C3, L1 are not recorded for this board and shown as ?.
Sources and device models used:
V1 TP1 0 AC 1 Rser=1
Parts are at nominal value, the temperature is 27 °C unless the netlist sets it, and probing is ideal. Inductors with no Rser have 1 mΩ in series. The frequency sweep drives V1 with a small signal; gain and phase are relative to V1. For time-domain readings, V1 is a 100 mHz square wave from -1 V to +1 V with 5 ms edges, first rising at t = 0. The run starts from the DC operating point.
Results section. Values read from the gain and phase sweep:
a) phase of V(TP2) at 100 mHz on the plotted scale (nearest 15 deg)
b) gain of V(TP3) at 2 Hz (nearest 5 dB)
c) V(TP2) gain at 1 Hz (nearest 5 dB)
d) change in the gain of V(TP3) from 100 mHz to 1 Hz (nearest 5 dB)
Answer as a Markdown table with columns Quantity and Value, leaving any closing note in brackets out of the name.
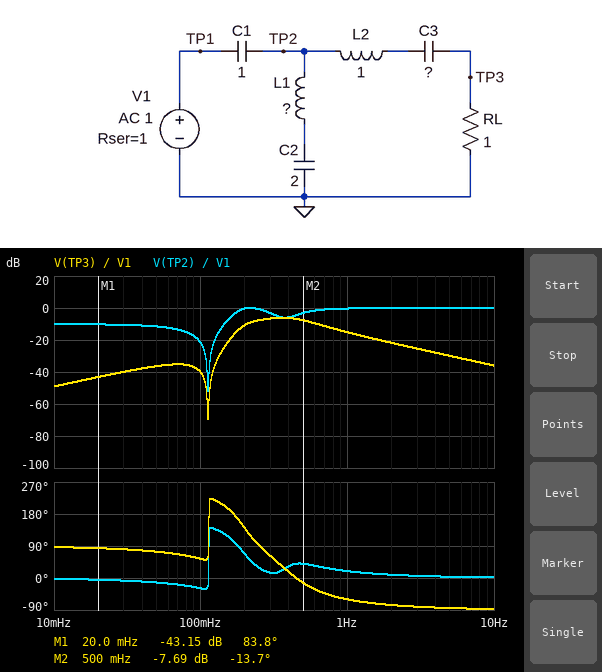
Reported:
| Quantity | Value |
|---|---|
| phase of V(TP2) at 100 mHz on the plotted scale | -30 deg |
| gain of V(TP3) at 2 Hz | -20 dB |
| V(TP2) gain at 1 Hz | 0 dB |
| change in the gain of V(TP3) from 100 mHz to 1 Hz | 25 dB |
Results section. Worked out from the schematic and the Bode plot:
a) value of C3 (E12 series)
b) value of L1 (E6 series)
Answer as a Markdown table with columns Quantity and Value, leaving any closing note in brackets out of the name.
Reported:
| Quantity | Value |
|---|---|
| value of C3 | 180 mF |
| value of L1 | 1 H |
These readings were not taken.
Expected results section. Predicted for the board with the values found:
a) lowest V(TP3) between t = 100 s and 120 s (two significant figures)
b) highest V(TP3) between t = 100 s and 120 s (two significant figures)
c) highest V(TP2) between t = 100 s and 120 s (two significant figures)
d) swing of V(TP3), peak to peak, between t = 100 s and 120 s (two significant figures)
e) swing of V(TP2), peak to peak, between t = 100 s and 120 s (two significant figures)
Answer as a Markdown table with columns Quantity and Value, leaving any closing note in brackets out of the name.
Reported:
| Quantity | Value |
|---|---|
| lowest V(TP3) between t = 100 s and 120 s | -390 mV |
| highest V(TP3) between t = 100 s and 120 s | 390 mV |
| highest V(TP2) between t = 100 s and 120 s | 1.8 V |
| swing of V(TP3), peak to peak, between t = 100 s and 120 s | 780 mV |
| swing of V(TP2), peak to peak, between t = 100 s and 120 s | 2.9 V |
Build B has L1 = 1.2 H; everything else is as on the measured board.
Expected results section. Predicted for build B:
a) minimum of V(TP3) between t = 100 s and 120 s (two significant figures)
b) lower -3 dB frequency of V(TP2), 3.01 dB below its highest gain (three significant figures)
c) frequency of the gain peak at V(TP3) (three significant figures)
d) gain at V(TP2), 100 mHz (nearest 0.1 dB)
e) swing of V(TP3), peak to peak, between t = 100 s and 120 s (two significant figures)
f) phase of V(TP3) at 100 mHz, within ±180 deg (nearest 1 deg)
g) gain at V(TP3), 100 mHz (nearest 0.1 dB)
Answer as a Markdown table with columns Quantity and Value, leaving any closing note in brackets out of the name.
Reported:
| Quantity | Value |
|---|---|
| minimum of V(TP3) between t = 100 s and 120 s | -380 mV |
| lower -3 dB frequency of V(TP2), 3.01 dB below its highest gain | 159 mHz |
| frequency of the gain peak at V(TP3) | 374 mHz |
| gain at V(TP2), 100 mHz | -33.3 dB |
| swing of V(TP3), peak to peak, between t = 100 s and 120 s | 760 mV |
| phase of V(TP3) at 100 mHz, within ±180 deg | 53 deg |
| gain at V(TP3), 100 mHz | -51.6 dB |
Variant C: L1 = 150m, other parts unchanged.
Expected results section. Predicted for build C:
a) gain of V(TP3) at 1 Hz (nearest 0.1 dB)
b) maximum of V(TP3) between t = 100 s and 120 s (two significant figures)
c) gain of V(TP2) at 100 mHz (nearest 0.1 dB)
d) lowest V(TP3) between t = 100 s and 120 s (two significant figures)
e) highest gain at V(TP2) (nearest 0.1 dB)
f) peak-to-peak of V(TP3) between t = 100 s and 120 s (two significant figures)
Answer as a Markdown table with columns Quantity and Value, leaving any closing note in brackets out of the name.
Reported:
| Quantity | Value |
|---|---|
| gain of V(TP3) at 1 Hz | -18.7 dB |
| maximum of V(TP3) between t = 100 s and 120 s | 150 mV |
| gain of V(TP2) at 100 mHz | -11.6 dB |
| lowest V(TP3) between t = 100 s and 120 s | -150 mV |
| highest gain at V(TP2) | 0 dB |
| peak-to-peak of V(TP3) between t = 100 s and 120 s | 310 mV |
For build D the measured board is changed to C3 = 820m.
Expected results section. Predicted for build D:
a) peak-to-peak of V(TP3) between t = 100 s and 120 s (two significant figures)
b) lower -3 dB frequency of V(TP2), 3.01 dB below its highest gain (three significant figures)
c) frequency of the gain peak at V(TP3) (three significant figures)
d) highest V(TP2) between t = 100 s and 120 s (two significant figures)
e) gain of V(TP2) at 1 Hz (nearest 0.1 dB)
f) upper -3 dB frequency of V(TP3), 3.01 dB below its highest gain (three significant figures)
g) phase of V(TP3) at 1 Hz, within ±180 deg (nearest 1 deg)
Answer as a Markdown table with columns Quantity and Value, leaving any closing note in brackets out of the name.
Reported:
| Quantity | Value |
|---|---|
| peak-to-peak of V(TP3) between t = 100 s and 120 s | 650 mV |
| lower -3 dB frequency of V(TP2), 3.01 dB below its highest gain | 333 mHz |
| frequency of the gain peak at V(TP3) | 233 mHz |
| highest V(TP2) between t = 100 s and 120 s | 1.9 V |
| gain of V(TP2) at 1 Hz | -0.2 dB |
| upper -3 dB frequency of V(TP3), 3.01 dB below its highest gain | 499 mHz |
| phase of V(TP3) at 1 Hz, within ±180 deg | -62 deg |
